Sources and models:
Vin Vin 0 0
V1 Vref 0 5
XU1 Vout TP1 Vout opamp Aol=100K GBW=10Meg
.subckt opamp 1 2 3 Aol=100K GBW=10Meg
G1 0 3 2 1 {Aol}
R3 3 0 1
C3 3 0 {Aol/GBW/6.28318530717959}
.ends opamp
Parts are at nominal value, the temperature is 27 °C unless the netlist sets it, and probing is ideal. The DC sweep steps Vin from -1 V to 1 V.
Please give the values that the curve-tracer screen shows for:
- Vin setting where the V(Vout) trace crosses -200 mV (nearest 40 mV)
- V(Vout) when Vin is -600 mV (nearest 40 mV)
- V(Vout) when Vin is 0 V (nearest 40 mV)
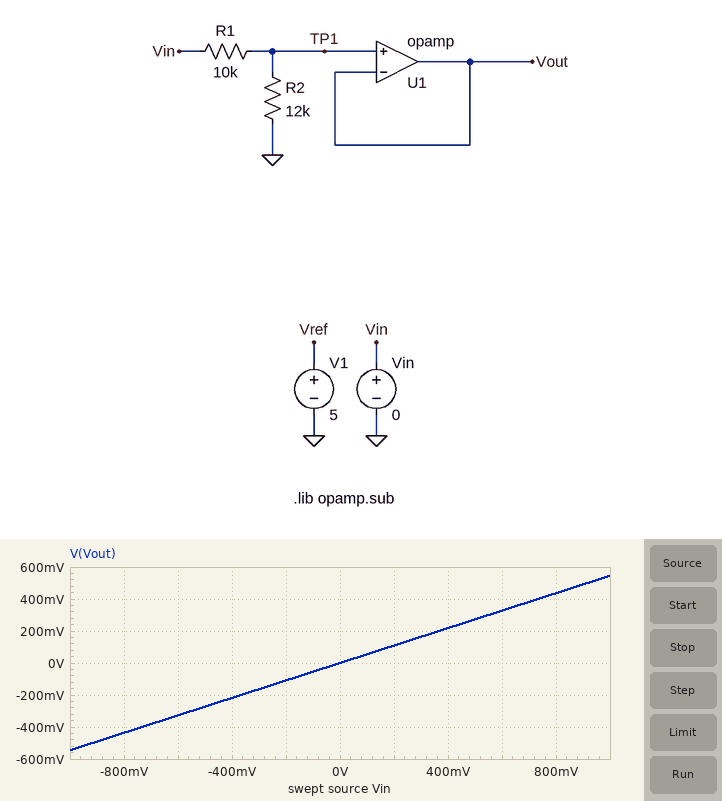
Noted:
-360 mV
-320 mV
0 V
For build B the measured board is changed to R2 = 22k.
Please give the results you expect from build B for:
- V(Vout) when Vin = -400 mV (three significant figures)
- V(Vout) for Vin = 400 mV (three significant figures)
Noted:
-275 mV
275 mV
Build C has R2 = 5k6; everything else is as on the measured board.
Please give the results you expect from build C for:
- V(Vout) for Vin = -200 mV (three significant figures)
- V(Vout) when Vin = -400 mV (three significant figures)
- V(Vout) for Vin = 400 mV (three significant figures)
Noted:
-71.8 mV
-144 mV
144 mV
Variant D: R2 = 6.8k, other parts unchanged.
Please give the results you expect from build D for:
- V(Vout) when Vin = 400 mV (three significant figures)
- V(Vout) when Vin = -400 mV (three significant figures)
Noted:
162 mV
-162 mV
